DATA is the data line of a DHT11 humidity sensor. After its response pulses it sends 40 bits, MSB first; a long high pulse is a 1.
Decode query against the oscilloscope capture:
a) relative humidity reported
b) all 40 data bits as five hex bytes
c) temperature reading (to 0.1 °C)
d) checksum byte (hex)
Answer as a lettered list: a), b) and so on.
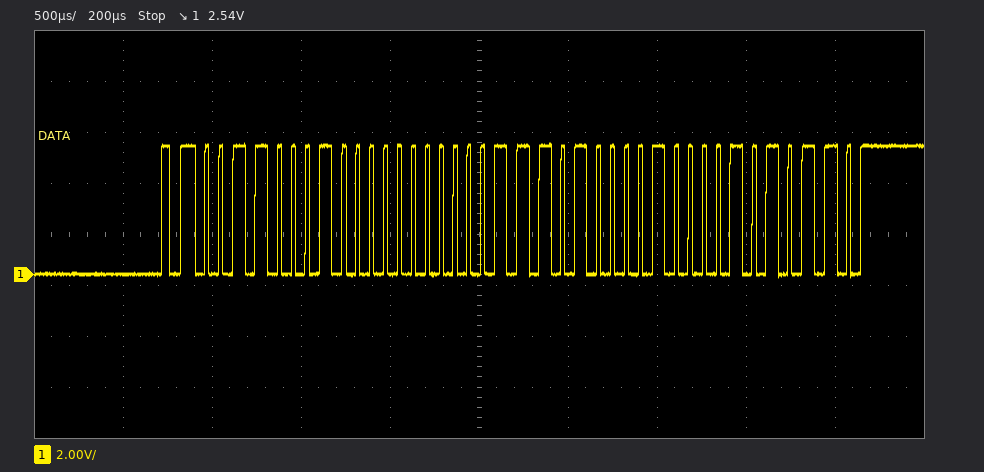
a) 49 %
b) 31 00 1D 08 56
c) 29.8 °C
d) 0x56
